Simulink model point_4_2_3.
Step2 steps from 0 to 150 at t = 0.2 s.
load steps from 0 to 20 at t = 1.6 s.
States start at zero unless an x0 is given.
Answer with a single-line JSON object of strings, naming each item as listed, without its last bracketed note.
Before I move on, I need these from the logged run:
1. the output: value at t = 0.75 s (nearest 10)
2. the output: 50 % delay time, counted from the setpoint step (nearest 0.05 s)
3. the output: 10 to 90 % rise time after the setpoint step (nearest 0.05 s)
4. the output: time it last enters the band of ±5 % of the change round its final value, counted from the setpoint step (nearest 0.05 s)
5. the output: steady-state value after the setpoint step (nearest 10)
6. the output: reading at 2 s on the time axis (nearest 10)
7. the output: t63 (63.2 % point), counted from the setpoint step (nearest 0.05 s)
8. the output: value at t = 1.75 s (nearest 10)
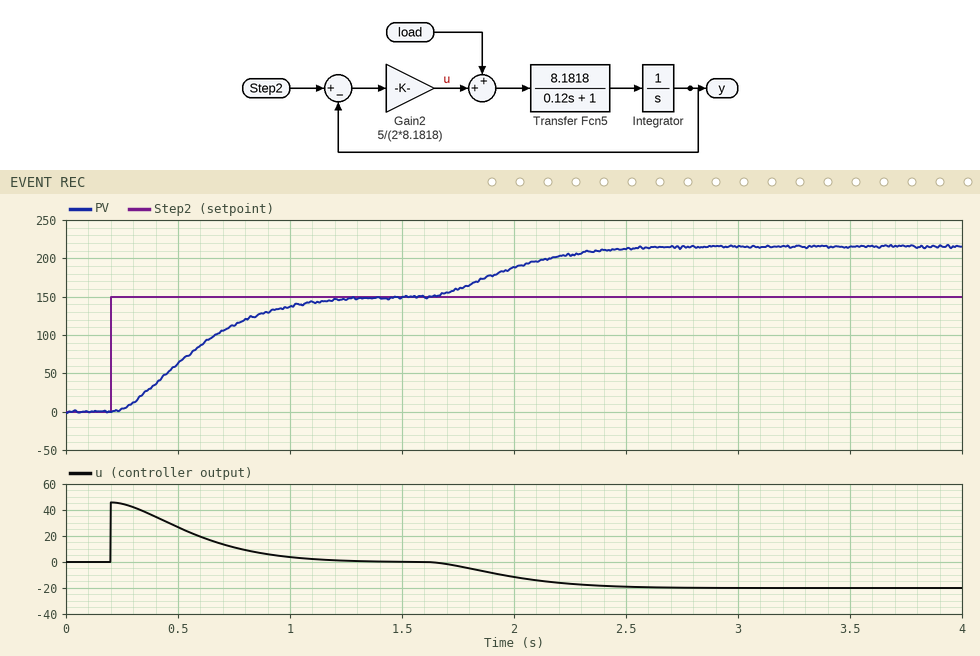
{"the output: value at t = 0.75 s": "110", "the output: 50 % delay time, counted from the setpoint step": "0.35 s", "the output: 10 to 90 % rise time after the setpoint step": "0.65 s", "the output: time it last enters the band of ±5 % of the change round its final value, counted from the setpoint step": "0.90 s", "the output: steady-state value after the setpoint step": "150", "the output: reading at 2 s on the time axis": "190", "the output: t63 (63.2 % point), counted from the setpoint step": "0.45 s", "the output: value at t = 1.75 s": "160"}
